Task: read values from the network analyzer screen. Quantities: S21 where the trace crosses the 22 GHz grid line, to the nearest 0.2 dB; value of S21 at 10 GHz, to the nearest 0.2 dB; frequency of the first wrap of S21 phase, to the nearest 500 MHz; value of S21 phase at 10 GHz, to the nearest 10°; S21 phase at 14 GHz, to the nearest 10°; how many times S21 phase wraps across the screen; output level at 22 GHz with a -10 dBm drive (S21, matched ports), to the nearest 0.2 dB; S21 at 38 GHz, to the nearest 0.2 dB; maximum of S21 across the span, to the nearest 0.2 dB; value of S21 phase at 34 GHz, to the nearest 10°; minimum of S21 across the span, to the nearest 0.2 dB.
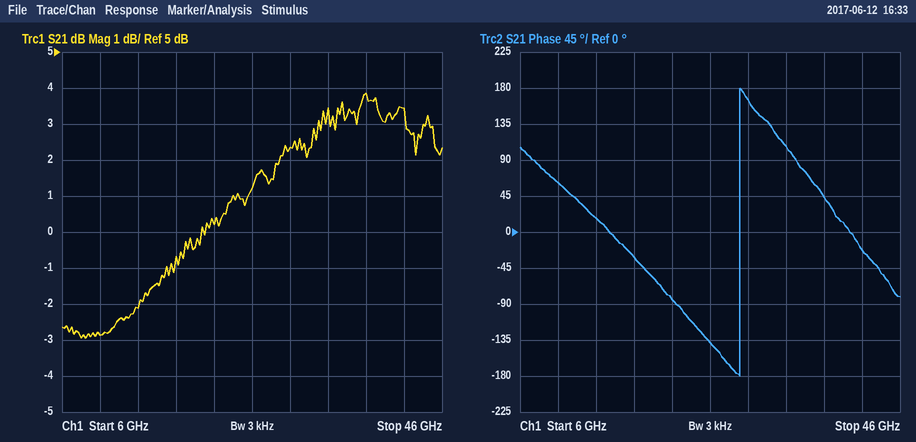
0.2 dB
-2.8 dB
29.0 GHz
60°
20°
1
-9.8 dBm
3.8 dB
3.8 dB
110°
-3.0 dB
